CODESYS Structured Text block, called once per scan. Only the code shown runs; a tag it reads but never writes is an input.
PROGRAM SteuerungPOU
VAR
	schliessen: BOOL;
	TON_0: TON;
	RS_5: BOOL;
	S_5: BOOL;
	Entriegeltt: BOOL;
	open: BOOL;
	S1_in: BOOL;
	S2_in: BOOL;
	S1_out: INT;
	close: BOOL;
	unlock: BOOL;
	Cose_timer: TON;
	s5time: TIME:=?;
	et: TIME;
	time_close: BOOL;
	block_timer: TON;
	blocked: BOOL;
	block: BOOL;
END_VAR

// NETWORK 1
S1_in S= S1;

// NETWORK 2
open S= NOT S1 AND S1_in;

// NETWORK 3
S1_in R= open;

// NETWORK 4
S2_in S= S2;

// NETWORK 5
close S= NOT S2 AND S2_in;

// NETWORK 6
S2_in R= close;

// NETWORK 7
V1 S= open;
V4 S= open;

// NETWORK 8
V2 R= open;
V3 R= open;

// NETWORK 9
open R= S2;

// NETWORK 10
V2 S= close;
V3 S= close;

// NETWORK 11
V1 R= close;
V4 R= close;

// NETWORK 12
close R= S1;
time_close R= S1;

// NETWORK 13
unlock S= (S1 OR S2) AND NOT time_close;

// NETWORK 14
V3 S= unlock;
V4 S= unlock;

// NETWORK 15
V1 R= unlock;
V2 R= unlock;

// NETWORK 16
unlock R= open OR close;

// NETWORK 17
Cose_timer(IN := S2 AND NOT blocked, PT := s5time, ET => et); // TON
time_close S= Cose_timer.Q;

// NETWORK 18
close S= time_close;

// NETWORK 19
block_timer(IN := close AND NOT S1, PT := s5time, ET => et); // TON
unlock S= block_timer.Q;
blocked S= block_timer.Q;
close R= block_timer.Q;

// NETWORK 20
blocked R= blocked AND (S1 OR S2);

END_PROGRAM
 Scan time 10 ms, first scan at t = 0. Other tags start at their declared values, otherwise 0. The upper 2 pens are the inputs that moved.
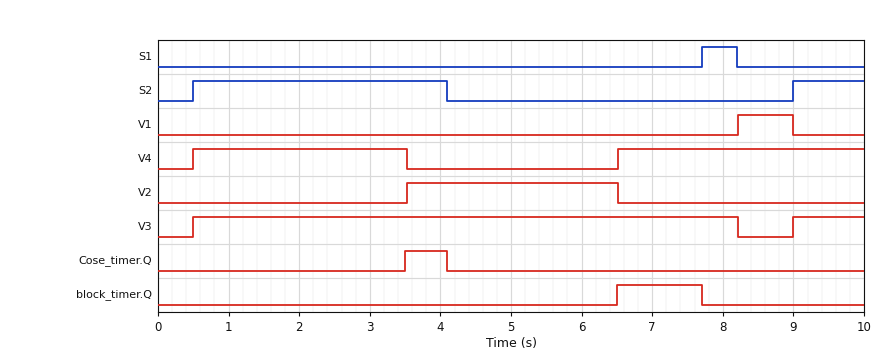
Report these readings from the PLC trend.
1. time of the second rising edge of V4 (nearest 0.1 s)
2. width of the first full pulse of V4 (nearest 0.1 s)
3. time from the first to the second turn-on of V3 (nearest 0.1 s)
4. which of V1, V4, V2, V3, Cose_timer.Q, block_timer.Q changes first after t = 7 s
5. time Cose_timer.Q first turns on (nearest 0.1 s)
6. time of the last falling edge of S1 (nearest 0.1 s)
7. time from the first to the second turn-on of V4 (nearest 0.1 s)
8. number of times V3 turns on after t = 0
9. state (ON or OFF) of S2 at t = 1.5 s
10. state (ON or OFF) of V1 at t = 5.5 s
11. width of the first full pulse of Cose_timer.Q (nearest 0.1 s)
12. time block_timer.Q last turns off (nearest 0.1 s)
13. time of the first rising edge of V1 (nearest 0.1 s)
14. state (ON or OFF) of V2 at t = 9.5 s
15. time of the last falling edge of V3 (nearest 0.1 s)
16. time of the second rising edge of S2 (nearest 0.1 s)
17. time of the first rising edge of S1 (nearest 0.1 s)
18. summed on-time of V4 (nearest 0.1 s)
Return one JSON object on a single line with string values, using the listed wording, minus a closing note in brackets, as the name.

{"time of the second rising edge of V4": "6.5 s", "width of the first full pulse of V4": "3.0 s", "time from the first to the second turn-on of V3": "8.5 s", "which of V1, V4, V2, V3, Cose_timer.Q, block_timer.Q changes first after t = 7 s": "block_timer.Q", "time Cose_timer.Q first turns on": "3.5 s", "time of the last falling edge of S1": "8.2 s", "time from the first to the second turn-on of V4": "6.0 s", "number of times V3 turns on after t = 0": "2", "state (ON or OFF) of S2 at t = 1.5 s": "ON", "state (ON or OFF) of V1 at t = 5.5 s": "OFF", "width of the first full pulse of Cose_timer.Q": "0.6 s", "time block_timer.Q last turns off": "7.7 s", "time of the first rising edge of V1": "8.2 s", "state (ON or OFF) of V2 at t = 9.5 s": "OFF", "time of the last falling edge of V3": "8.2 s", "time of the second rising edge of S2": "9.0 s", "time of the first rising edge of S1": "7.7 s", "summed on-time of V4": "6.5 s"}
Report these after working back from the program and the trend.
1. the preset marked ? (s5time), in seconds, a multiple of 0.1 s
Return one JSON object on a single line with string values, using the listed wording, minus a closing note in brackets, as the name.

{"the preset marked ? (s5time), in seconds, a multiple of 0.1 s": "3.0 s"}
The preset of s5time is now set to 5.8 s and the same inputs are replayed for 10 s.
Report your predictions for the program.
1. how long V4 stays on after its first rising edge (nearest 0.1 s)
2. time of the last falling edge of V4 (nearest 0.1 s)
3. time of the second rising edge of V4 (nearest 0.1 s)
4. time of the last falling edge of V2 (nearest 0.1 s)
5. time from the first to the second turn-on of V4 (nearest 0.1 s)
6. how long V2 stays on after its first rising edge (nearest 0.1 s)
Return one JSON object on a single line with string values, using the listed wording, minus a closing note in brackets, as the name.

{"how long V4 stays on after its first rising edge": "3.6 s", "time of the last falling edge of V4": "4.1 s", "time of the second rising edge of V4": "7.7 s", "time of the last falling edge of V2": "7.7 s", "time from the first to the second turn-on of V4": "7.2 s", "how long V2 stays on after its first rising edge": "3.6 s"}
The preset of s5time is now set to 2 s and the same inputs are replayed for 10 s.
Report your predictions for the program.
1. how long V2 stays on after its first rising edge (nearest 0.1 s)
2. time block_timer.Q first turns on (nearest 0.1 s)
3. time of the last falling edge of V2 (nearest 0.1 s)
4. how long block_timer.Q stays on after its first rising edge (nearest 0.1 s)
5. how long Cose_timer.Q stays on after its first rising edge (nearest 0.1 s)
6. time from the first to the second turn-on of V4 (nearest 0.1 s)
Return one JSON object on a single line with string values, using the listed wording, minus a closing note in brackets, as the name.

{"how long V2 stays on after its first rising edge": "2.0 s", "time block_timer.Q first turns on": "4.5 s", "time of the last falling edge of V2": "4.5 s", "how long block_timer.Q stays on after its first rising edge": "3.2 s", "how long Cose_timer.Q stays on after its first rising edge": "1.6 s", "time from the first to the second turn-on of V4": "4.0 s"}
